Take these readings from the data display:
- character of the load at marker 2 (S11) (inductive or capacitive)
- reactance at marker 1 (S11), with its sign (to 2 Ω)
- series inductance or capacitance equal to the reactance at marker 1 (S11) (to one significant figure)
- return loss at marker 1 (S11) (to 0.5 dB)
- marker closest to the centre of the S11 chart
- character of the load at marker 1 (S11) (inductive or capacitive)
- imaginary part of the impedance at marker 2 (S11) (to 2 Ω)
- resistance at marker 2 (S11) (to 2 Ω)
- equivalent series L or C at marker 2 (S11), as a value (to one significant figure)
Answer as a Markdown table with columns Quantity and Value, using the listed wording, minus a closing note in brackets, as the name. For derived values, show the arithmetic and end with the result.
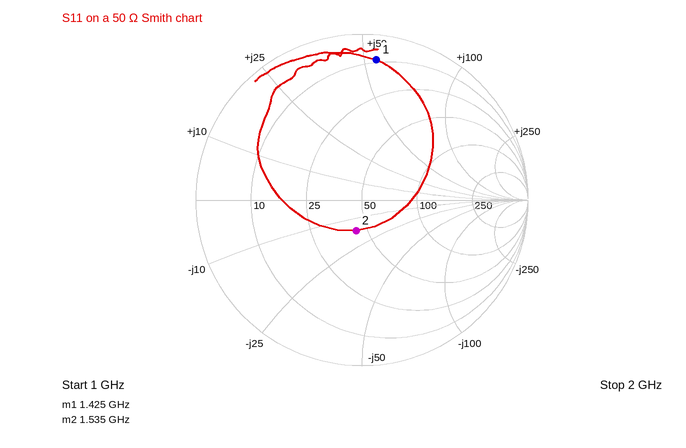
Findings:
| Quantity | Value |
|---|---|
| character of the load at marker 2 (S11) | capacitive |
| reactance at marker 1 (S11), with its sign | +54 Ω |
| series inductance or capacitance equal to the reactance at marker 1 (S11) | L = 54 Ω/(2π × 1.425 GHz) ≈ 6 nH |
| return loss at marker 1 (S11) | 1.5 dB |
| marker closest to the centre of the S11 chart | marker 2 |
| character of the load at marker 1 (S11) | inductive |
| imaginary part of the impedance at marker 2 (S11) | -16 Ω |
| resistance at marker 2 (S11) | 44 Ω |
| equivalent series L or C at marker 2 (S11), as a value | C = 1/(2π × 1.535 GHz × 16 Ω) ≈ 6 pF |
